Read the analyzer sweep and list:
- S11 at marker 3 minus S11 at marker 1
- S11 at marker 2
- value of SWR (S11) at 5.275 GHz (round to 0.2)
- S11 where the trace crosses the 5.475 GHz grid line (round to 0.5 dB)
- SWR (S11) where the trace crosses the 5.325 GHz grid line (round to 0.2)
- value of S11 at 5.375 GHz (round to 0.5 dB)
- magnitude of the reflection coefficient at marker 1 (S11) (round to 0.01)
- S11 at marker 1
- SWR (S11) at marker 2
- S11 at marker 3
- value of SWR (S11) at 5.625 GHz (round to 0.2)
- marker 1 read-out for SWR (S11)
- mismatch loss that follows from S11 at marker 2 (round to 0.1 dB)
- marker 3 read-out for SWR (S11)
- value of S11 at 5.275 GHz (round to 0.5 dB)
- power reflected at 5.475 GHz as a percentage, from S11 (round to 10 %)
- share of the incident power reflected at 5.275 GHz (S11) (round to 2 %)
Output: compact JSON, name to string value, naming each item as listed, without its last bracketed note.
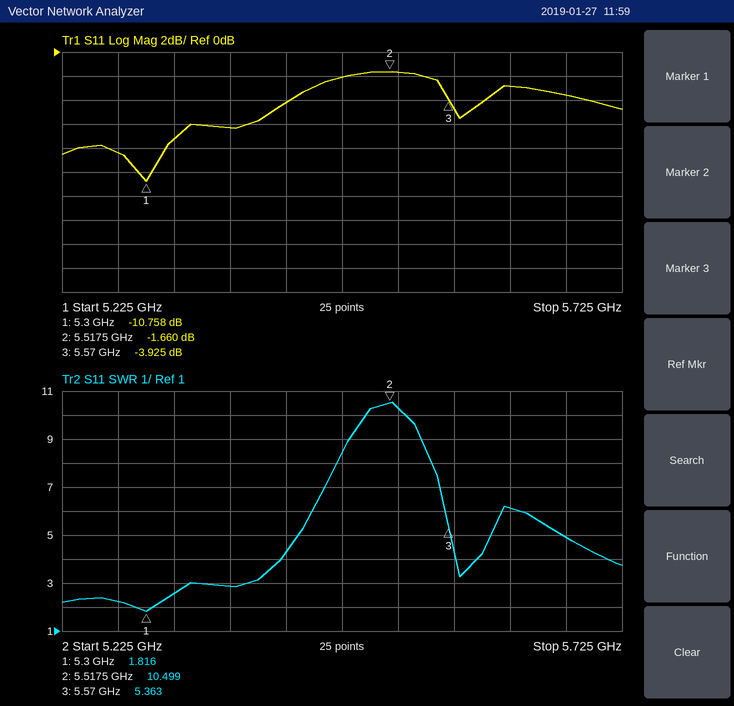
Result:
{"S11 at marker 3 minus S11 at marker 1": "6.833 dB", "S11 at marker 2": "-1.660 dB", "value of SWR (S11) at 5.275 GHz": "2.2", "S11 where the trace crosses the 5.475 GHz grid line": "-2.0 dB", "SWR (S11) where the trace crosses the 5.325 GHz grid line": "2.6", "value of S11 at 5.375 GHz": "-6.5 dB", "magnitude of the reflection coefficient at marker 1 (S11)": "0.29", "S11 at marker 1": "-10.758 dB", "SWR (S11) at marker 2": "10.499", "S11 at marker 3": "-3.925 dB", "value of SWR (S11) at 5.625 GHz": "6.2", "marker 1 read-out for SWR": "1.816", "mismatch loss that follows from S11 at marker 2": "5.0 dB", "marker 3 read-out for SWR": "5.363", "value of S11 at 5.275 GHz": "-8.5 dB", "power reflected at 5.475 GHz as a percentage, from S11": "60 %", "share of the incident power reflected at 5.275 GHz (S11)": "14 %"}
